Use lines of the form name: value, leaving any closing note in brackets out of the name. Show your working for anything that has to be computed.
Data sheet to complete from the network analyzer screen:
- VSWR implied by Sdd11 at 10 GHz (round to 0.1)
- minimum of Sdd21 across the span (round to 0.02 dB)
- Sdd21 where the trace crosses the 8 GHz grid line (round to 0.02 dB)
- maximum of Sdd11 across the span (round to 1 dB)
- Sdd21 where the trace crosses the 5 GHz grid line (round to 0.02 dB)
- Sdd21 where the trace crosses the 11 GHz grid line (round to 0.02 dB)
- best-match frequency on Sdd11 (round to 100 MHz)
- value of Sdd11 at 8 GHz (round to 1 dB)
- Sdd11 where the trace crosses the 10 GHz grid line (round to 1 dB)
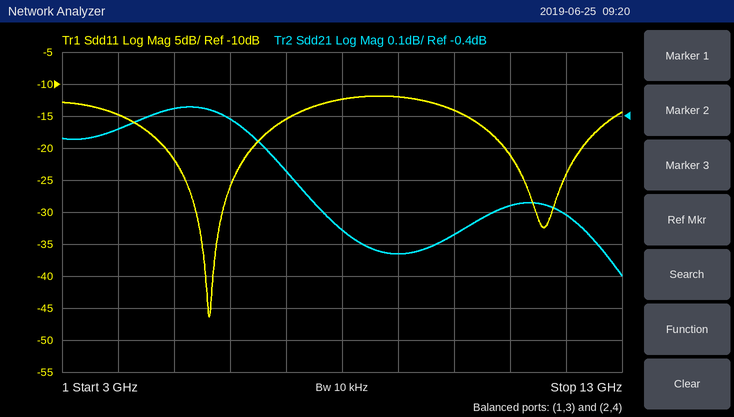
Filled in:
VSWR implied by Sdd11 at 10 GHz: |Γ| = 10^(-14/20) = 0.1995; VSWR = (1 + 0.1995)/(1 − 0.1995) ≈ 1.5
minimum of Sdd21 across the span: -0.90 dB
Sdd21 where the trace crosses the 8 GHz grid line: -0.76 dB
maximum of Sdd11 across the span: -12 dB
Sdd21 where the trace crosses the 5 GHz grid line: -0.38 dB
Sdd21 where the trace crosses the 11 GHz grid line: -0.68 dB
best-match frequency on Sdd11: 5.6 GHz
value of Sdd11 at 8 GHz: -12 dB
Sdd11 where the trace crosses the 10 GHz grid line: -14 dB
